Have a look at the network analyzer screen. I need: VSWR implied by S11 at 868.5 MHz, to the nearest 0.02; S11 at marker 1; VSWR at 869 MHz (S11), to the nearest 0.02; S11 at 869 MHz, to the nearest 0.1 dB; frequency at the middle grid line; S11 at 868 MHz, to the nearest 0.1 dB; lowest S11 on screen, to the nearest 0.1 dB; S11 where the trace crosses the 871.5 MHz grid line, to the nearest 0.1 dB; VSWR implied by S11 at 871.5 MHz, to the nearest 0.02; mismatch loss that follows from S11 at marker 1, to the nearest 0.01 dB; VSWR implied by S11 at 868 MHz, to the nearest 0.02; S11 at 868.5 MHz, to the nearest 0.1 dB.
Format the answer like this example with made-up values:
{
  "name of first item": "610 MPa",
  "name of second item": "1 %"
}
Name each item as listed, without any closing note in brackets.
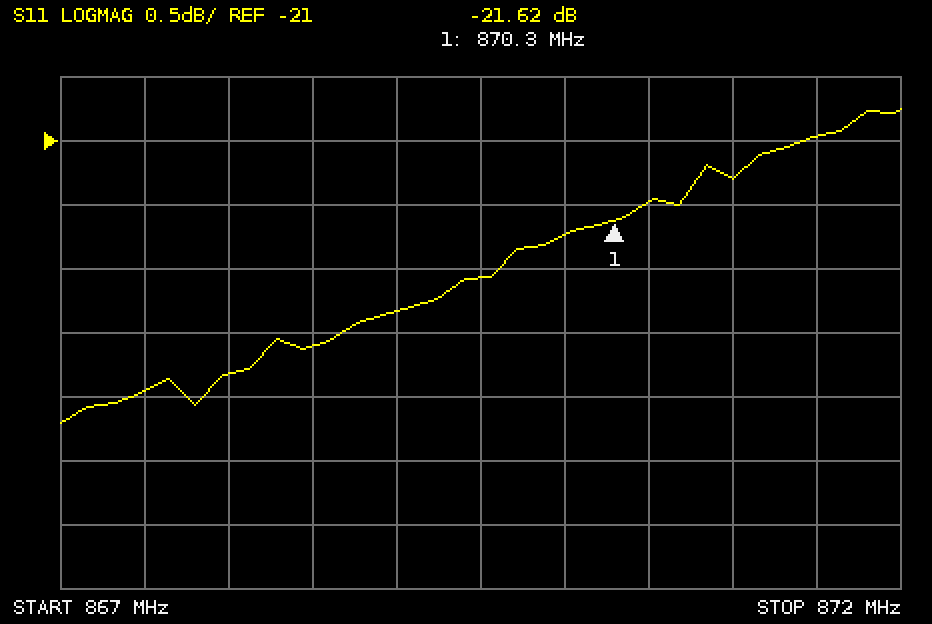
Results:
{
  "VSWR implied by S11 at 868.5 MHz, to the nearest 0.02": "1.16",
  "S11 at marker 1": "-21.62 dB",
  "VSWR at 869 MHz (S11), to the nearest 0.02": "1.16",
  "S11 at 869 MHz, to the nearest 0.1 dB": "-22.3 dB",
  "frequency at the middle grid line": "869.5 MHz",
  "S11 at 868 MHz, to the nearest 0.1 dB": "-22.8 dB",
  "lowest S11 on screen, to the nearest 0.1 dB": "-23.2 dB",
  "S11 where the trace crosses the 871.5 MHz grid line, to the nearest 0.1 dB": "-21.0 dB",
  "VSWR implied by S11 at 871.5 MHz, to the nearest 0.02": "1.20",
  "mismatch loss that follows from S11 at marker 1, to the nearest 0.01 dB": "0.03 dB",
  "VSWR implied by S11 at 868 MHz, to the nearest 0.02": "1.16",
  "S11 at 868.5 MHz, to the nearest 0.1 dB": "-22.6 dB"
}
